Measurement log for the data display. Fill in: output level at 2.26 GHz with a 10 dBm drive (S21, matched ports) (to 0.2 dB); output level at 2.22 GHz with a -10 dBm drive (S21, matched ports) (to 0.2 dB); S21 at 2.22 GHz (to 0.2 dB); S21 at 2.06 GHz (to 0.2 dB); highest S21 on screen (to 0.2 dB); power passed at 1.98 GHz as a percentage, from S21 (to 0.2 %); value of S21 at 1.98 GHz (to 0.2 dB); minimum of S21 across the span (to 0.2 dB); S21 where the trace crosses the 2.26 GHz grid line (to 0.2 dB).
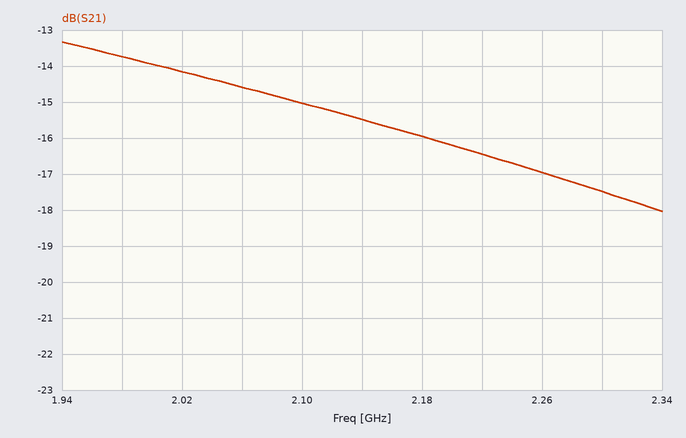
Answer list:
-7.0 dBm
-26.4 dBm
-16.4 dB
-14.6 dB
-13.4 dB
4.2 %
-13.8 dB
-18.0 dB
-17.0 dB
